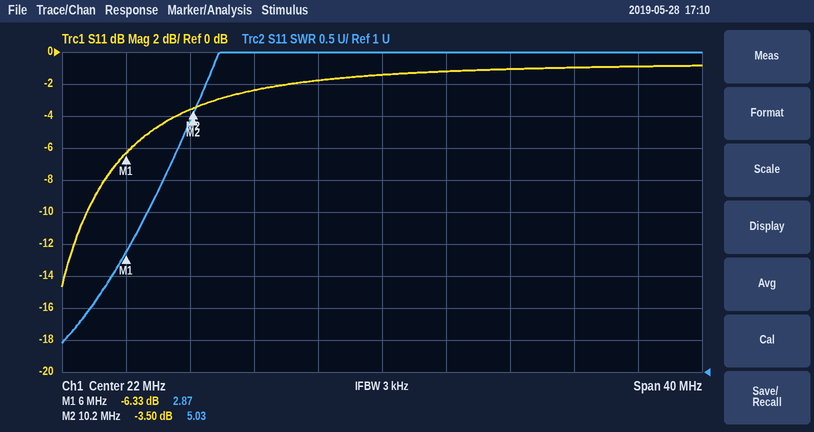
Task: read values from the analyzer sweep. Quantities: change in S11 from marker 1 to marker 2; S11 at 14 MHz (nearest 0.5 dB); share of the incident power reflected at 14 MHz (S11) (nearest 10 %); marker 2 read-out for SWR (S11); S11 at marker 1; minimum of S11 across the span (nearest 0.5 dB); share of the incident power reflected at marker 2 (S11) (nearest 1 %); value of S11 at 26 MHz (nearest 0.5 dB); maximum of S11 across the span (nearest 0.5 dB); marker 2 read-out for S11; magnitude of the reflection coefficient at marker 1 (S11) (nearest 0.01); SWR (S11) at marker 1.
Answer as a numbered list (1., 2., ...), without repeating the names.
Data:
1. 2.83 dB
2. -2.5 dB
3. 60 %
4. 5.03
5. -6.33 dB
6. -14.5 dB
7. 45 %
8. -1.0 dB
9. -1.0 dB
10. -3.50 dB
11. 0.48
12. 2.87
